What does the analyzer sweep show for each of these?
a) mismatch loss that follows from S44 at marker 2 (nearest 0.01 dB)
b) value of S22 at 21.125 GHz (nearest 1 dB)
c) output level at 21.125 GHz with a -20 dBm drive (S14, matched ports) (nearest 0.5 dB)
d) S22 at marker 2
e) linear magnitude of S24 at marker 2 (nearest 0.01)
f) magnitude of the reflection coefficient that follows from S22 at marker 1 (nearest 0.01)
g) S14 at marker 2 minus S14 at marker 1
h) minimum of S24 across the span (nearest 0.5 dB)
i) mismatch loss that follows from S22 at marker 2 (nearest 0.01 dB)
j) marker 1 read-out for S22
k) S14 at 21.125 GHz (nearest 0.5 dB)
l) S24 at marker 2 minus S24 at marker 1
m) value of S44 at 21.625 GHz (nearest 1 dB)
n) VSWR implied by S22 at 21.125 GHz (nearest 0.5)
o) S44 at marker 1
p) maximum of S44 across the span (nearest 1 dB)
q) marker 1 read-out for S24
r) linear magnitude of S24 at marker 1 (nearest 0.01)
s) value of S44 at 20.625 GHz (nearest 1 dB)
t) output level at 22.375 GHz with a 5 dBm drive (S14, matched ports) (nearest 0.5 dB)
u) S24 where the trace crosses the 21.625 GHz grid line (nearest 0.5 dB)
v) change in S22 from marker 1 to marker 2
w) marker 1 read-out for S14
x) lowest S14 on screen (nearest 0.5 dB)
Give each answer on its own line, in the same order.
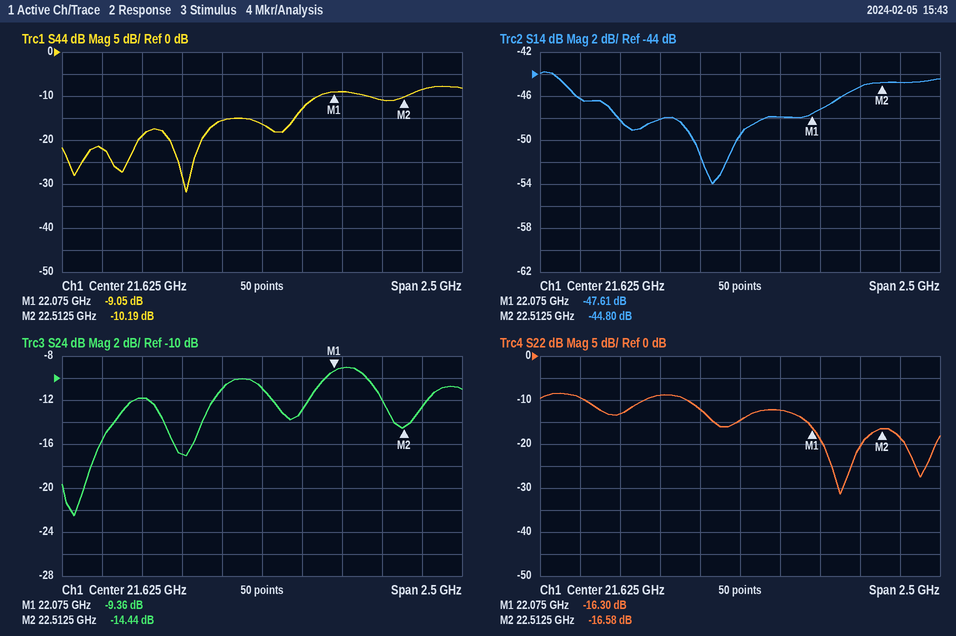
0.44 dB
-9 dB
-68.0 dBm
-16.58 dB
0.19
0.15
2.81 dB
-22.5 dB
0.10 dB
-16.30 dB
-48.0 dB
-5.08 dB
-16 dB
2.0
-9.05 dB
-8 dB
-9.36 dB
0.34
-22 dB
-40.0 dBm
-11.0 dB
-0.28 dB
-47.61 dB
-54.0 dB
